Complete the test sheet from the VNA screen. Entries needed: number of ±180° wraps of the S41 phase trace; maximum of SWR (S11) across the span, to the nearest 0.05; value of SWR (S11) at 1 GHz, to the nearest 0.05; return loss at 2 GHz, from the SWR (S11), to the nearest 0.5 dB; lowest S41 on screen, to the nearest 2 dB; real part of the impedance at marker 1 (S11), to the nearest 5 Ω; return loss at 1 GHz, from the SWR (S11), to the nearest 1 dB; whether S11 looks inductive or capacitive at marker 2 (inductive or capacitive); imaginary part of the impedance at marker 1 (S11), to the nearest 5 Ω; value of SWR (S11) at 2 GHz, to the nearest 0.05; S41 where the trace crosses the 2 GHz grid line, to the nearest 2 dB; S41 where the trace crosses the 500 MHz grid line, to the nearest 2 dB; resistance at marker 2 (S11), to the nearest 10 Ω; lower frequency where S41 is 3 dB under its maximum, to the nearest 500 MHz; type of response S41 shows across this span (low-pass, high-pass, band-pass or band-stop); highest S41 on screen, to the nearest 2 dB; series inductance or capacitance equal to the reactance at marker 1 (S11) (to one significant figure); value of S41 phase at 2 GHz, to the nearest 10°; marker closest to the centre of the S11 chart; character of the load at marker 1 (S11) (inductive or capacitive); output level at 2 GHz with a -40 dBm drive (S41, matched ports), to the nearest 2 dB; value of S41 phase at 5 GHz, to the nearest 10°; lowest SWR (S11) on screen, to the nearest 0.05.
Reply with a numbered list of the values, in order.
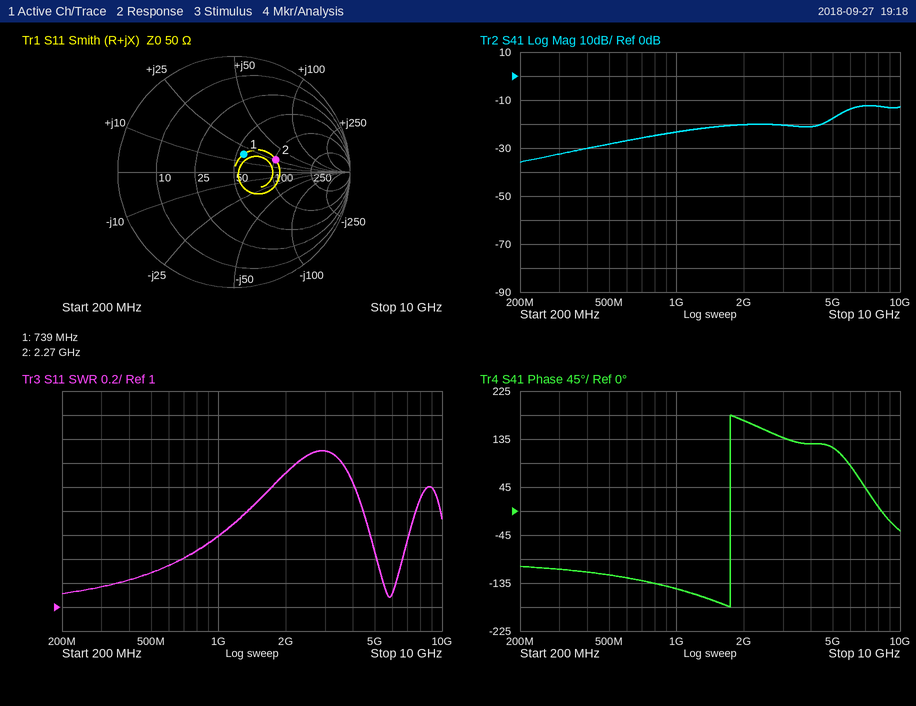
1. 1
2. 2.30
3. 1.60
4. 9.0 dB
5. -36 dB
6. 55 Ω
7. 13 dB
8. inductive
9. +20 Ω
10. 2.10
11. -20 dB
12. -28 dB
13. 100 Ω
14. 5.5 GHz
15. high-pass
16. -12 dB
17. 4 nH
18. 170°
19. marker 1
20. inductive
21. -60 dBm
22. 120°
23. 1.10
